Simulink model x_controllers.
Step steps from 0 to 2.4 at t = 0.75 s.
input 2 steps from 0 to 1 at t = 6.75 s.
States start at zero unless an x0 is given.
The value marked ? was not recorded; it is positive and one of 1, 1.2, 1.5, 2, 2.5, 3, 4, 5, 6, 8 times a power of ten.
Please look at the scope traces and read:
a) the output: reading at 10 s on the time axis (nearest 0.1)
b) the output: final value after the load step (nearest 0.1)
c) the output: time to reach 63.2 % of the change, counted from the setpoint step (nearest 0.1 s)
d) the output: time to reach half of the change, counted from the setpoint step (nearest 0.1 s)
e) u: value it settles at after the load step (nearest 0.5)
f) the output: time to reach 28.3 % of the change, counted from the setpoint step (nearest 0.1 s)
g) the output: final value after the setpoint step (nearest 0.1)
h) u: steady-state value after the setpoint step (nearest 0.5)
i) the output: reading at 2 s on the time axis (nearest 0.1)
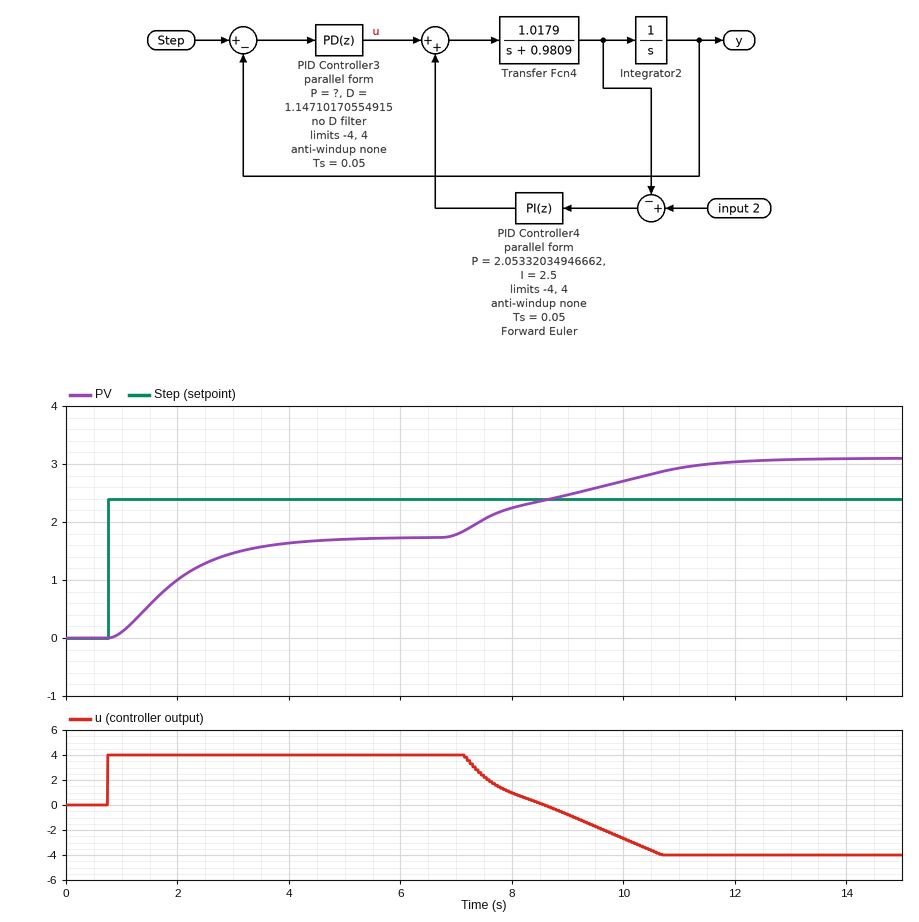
2.7
3.1
1.4 s
1.1 s
-4.0
0.7 s
1.7
4.0
1.0
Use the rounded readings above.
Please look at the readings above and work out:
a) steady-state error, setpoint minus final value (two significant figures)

0.70
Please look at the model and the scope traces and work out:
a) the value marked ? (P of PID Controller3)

8
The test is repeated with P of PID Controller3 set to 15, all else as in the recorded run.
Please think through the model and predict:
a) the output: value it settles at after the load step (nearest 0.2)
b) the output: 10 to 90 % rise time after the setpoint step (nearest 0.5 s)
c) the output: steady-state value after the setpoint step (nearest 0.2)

2.8
2.5 s
1.8
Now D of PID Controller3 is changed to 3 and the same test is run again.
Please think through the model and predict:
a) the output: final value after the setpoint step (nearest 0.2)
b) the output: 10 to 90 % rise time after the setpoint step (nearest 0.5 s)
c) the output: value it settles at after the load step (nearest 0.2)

1.8
2.5 s
3.0
